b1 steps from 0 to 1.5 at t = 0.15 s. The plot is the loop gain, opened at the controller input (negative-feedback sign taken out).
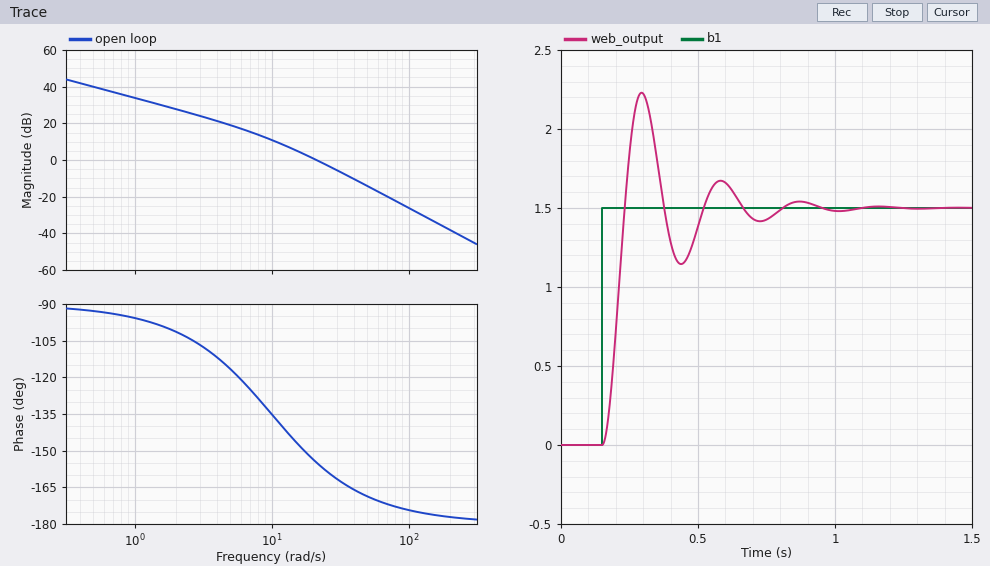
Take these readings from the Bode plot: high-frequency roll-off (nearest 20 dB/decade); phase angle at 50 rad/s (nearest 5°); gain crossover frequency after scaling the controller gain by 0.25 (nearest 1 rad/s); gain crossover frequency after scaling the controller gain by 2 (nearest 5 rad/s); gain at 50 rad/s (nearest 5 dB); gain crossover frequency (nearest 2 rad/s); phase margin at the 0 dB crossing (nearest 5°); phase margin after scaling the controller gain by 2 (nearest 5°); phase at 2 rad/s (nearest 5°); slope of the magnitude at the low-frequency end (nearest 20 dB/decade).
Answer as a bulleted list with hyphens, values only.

- -40 dB/decade
- -170°
- 9 rad/s
- 30 rad/s
- -15 dB
- 22 rad/s
- 25°
- 20°
- -100°
- -20 dB/decade
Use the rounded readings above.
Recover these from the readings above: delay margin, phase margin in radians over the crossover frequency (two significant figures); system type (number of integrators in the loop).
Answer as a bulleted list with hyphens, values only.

- 0.020 s
- 1
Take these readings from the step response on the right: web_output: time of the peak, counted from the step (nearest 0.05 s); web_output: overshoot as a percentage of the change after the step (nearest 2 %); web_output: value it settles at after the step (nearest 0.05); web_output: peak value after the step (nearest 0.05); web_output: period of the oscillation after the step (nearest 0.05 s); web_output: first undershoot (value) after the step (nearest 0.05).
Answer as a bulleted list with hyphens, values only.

- 0.15 s
- 48 %
- 1.50
- 2.25
- 0.30 s
- 1.15
